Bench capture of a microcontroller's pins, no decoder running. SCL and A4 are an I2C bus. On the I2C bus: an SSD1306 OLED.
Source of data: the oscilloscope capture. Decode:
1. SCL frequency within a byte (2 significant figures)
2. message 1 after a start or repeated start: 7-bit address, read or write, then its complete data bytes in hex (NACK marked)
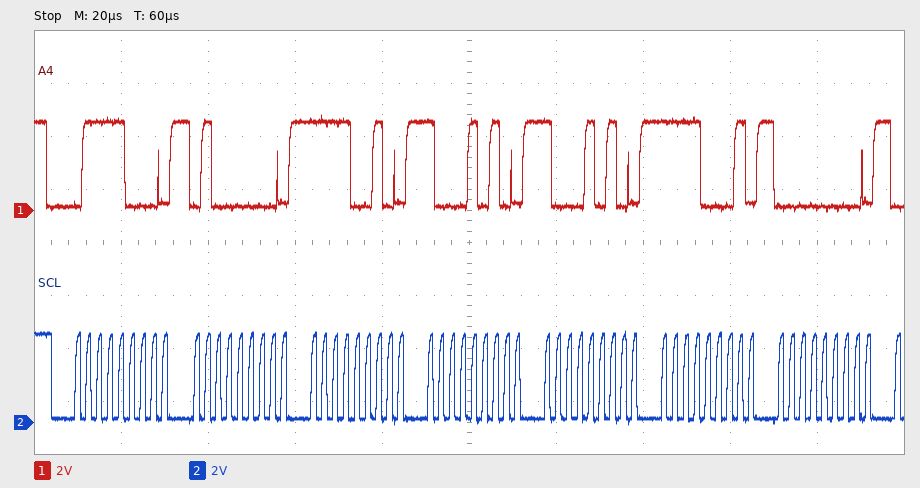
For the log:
400 kHz
0x3C write: 40 F2 8A 8A F1 00
